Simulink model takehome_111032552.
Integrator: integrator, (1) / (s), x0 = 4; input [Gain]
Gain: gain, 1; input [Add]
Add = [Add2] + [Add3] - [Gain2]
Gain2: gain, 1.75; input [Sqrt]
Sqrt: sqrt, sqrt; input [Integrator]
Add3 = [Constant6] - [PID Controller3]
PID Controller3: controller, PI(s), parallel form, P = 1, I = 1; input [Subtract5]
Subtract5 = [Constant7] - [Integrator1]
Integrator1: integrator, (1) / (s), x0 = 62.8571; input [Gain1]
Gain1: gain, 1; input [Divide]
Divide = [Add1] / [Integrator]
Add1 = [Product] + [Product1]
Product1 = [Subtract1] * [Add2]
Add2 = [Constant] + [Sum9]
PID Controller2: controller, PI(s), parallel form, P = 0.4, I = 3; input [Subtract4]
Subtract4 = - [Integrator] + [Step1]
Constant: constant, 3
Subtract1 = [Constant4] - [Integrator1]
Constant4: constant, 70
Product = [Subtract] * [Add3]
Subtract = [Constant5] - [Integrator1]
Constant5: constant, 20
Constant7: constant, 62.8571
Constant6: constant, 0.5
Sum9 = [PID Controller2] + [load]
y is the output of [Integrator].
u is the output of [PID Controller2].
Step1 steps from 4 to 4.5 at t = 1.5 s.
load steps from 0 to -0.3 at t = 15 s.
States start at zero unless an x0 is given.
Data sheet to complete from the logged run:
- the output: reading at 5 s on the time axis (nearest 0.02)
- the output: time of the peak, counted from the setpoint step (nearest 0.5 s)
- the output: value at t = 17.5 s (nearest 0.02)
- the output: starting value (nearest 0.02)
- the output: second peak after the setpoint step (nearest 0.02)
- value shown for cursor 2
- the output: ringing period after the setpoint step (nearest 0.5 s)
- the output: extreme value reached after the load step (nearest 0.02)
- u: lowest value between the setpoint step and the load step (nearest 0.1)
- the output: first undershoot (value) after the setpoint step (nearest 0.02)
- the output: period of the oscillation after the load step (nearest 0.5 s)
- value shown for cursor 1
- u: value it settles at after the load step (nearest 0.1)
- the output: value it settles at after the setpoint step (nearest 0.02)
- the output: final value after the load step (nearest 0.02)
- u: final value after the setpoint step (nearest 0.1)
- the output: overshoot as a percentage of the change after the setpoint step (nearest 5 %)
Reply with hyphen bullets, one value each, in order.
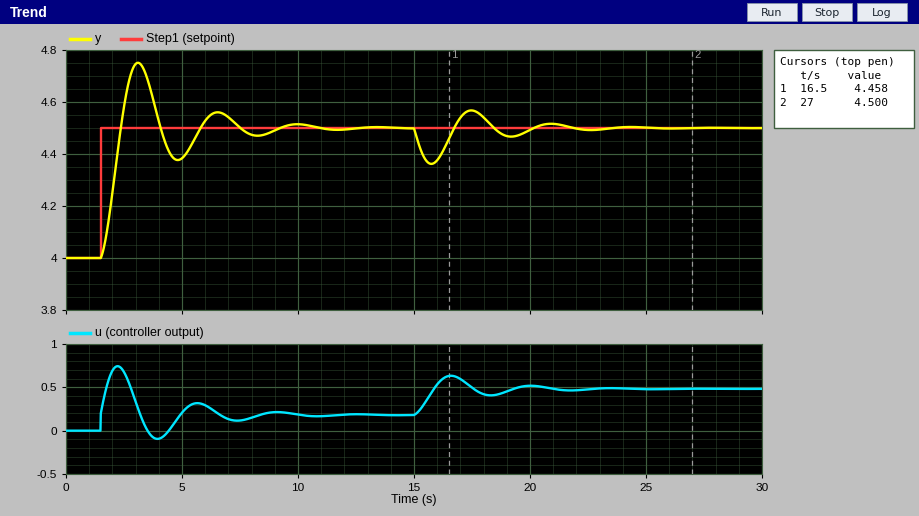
- 4.38
- 1.5 s
- 4.56
- 4.00
- 4.56
- 4.500
- 3.5 s
- 4.36
- -0.1
- 4.38
- 3.5 s
- 4.458
- 0.5
- 4.50
- 4.50
- 0.2
- 50 %
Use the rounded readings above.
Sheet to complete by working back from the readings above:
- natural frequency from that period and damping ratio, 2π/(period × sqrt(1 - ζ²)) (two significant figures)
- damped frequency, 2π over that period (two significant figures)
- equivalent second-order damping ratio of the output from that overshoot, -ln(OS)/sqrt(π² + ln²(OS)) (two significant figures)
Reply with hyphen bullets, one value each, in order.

- 1.8 rad/s
- 1.8 rad/s
- 0.22
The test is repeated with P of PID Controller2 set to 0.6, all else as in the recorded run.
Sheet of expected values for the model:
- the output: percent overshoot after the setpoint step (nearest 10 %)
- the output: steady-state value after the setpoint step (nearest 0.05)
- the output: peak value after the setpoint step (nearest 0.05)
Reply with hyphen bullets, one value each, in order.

- 40 %
- 4.50
- 4.70
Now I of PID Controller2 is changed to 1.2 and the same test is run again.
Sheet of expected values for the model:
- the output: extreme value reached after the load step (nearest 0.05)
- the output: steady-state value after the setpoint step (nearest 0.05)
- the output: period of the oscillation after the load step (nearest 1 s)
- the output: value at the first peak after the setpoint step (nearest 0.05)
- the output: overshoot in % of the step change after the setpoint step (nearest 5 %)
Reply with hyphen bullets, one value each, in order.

- 4.30
- 4.50
- 6 s
- 4.65
- 30 %
